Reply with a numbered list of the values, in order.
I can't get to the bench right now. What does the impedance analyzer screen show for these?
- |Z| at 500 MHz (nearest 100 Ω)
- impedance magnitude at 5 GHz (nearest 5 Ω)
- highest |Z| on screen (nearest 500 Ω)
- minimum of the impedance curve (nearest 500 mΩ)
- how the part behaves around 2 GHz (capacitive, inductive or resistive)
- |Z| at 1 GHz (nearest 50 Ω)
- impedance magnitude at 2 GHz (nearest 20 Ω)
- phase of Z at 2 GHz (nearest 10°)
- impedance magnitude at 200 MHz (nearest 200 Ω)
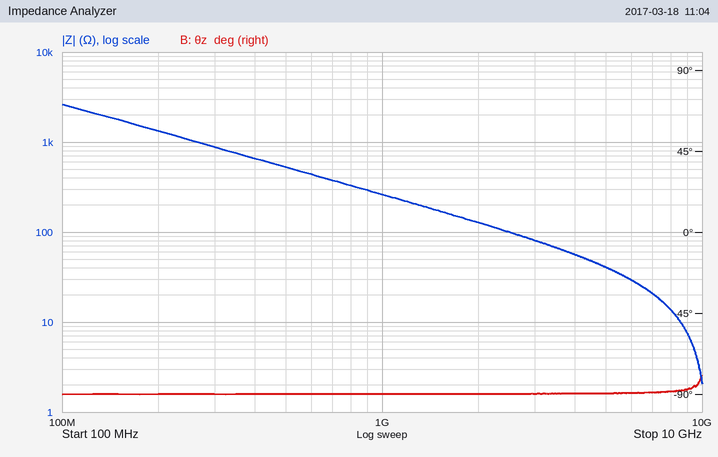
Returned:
1. 500 Ω
2. 40 Ω
3. 2.5 kΩ
4. 2.0 Ω
5. capacitive
6. 250 Ω
7. 120 Ω
8. -90°
9. 1.4 kΩ
